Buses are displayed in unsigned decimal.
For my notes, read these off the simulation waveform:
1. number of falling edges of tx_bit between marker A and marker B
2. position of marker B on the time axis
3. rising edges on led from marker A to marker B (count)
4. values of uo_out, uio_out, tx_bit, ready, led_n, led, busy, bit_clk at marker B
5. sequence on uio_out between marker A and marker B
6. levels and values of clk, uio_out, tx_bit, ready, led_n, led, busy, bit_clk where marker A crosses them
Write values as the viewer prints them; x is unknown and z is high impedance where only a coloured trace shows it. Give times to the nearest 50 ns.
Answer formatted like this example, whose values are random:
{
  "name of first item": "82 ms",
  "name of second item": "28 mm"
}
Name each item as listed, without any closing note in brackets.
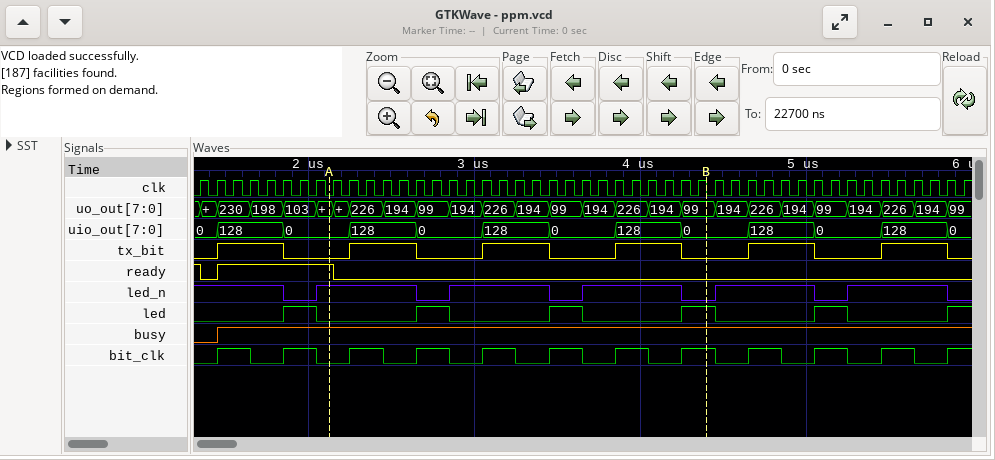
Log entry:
{
  "number of falling edges of tx_bit between marker A and marker B": "3",
  "position of marker B on the time axis": "4400 ns",
  "rising edges on led from marker A to marker B": "3",
  "values of uo_out, uio_out, tx_bit, ready, led_n, led, busy, bit_clk at marker B": "uo_out=99, uio_out=0, tx_bit=0, ready=0, led_n=0, led=1, busy=1, bit_clk=1",
  "sequence on uio_out between marker A and marker B": "0, 128, 0, 128, 0, 128, 0",
  "levels and values of clk, uio_out, tx_bit, ready, led_n, led, busy, bit_clk where marker A crosses them": "clk=0, uio_out=0, tx_bit=0, ready=1, led_n=1, led=0, busy=1, bit_clk=0"
}
